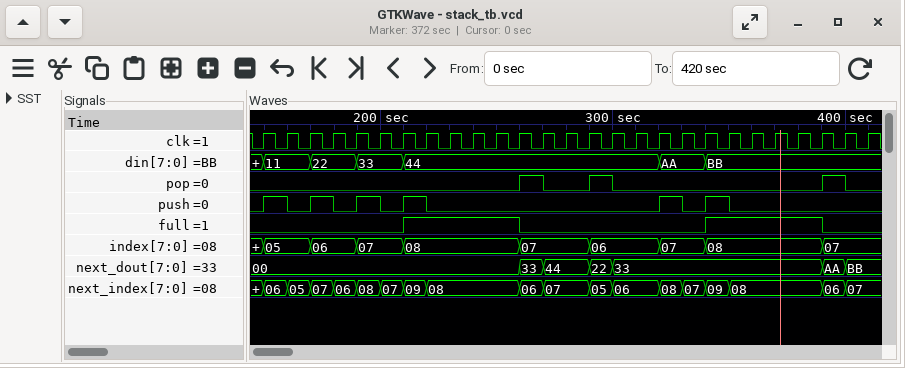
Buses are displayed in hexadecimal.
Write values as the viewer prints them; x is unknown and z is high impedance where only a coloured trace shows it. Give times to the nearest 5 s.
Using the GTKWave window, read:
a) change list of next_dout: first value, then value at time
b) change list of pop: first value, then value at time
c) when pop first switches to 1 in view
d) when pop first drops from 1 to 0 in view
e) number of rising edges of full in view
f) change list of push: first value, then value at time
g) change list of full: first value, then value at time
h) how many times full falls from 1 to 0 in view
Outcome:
00, 33 at 260 s, 44 at 270 s, 22 at 290 s, 33 at 300 s, AA at 390 s, BB at 400 s
0, 1 at 260 s, 0 at 270 s, 1 at 290 s, 0 at 300 s, 1 at 390 s, 0 at 400 s
260 s
270 s
2
0, 1 at 150 s, 0 at 160 s, 1 at 170 s, 0 at 180 s, 1 at 190 s, 0 at 200 s, 1 at 210 s, 0 at 220 s, 1 at 320 s, 0 at 330 s, 1 at 340 s, 0 at 350 s
0, 1 at 210 s, 0 at 260 s, 1 at 340 s, 0 at 390 s
2
